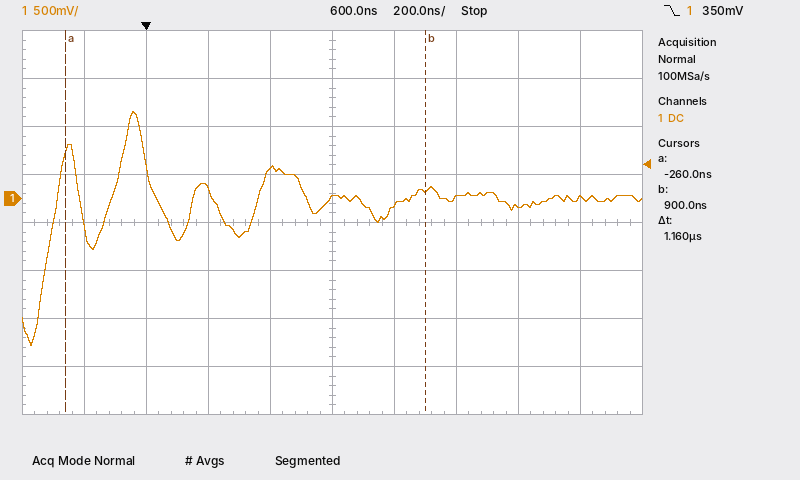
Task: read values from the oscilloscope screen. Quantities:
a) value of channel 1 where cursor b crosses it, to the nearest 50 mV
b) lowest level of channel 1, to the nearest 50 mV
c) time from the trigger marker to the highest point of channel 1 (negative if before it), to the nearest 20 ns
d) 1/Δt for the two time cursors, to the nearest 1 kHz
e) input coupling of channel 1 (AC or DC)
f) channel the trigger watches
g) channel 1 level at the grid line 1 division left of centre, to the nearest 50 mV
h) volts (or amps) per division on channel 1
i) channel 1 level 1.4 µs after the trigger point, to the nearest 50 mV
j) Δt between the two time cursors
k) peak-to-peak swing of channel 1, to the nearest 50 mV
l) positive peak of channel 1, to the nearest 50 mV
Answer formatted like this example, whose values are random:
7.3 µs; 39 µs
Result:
100 mV; -1.55 V; -40 ns; 862 kHz; DC; channel 1; 300 mV; 500 mV; 0 mV; 1.16 µs; 2.45 V; 900 mV
